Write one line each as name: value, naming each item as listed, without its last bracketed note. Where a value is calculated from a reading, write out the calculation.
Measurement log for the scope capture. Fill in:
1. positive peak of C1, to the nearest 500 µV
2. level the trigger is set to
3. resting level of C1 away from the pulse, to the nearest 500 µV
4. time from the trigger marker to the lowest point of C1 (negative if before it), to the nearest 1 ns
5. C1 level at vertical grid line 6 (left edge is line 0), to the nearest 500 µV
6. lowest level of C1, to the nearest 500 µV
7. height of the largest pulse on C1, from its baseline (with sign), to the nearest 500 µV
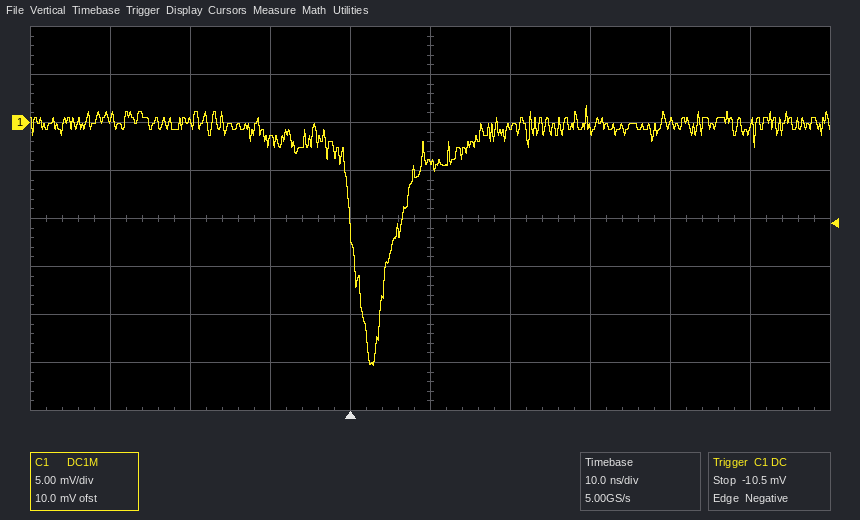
positive peak of C1, to the nearest 500 µV: 2.0 mV
level the trigger is set to: -10.5 mV
resting level of C1 away from the pulse, to the nearest 500 µV: -500 µV
time from the trigger marker to the lowest point of C1 (negative if before it), to the nearest 1 ns: +3 ns
C1 level at vertical grid line 6 (left edge is line 0), to the nearest 500 µV: -500 µV
lowest level of C1, to the nearest 500 µV: -25.5 mV
height of the largest pulse on C1, from its baseline (with sign), to the nearest 500 µV: -25.5 mV − (-500 µV) = -25.0 mV
